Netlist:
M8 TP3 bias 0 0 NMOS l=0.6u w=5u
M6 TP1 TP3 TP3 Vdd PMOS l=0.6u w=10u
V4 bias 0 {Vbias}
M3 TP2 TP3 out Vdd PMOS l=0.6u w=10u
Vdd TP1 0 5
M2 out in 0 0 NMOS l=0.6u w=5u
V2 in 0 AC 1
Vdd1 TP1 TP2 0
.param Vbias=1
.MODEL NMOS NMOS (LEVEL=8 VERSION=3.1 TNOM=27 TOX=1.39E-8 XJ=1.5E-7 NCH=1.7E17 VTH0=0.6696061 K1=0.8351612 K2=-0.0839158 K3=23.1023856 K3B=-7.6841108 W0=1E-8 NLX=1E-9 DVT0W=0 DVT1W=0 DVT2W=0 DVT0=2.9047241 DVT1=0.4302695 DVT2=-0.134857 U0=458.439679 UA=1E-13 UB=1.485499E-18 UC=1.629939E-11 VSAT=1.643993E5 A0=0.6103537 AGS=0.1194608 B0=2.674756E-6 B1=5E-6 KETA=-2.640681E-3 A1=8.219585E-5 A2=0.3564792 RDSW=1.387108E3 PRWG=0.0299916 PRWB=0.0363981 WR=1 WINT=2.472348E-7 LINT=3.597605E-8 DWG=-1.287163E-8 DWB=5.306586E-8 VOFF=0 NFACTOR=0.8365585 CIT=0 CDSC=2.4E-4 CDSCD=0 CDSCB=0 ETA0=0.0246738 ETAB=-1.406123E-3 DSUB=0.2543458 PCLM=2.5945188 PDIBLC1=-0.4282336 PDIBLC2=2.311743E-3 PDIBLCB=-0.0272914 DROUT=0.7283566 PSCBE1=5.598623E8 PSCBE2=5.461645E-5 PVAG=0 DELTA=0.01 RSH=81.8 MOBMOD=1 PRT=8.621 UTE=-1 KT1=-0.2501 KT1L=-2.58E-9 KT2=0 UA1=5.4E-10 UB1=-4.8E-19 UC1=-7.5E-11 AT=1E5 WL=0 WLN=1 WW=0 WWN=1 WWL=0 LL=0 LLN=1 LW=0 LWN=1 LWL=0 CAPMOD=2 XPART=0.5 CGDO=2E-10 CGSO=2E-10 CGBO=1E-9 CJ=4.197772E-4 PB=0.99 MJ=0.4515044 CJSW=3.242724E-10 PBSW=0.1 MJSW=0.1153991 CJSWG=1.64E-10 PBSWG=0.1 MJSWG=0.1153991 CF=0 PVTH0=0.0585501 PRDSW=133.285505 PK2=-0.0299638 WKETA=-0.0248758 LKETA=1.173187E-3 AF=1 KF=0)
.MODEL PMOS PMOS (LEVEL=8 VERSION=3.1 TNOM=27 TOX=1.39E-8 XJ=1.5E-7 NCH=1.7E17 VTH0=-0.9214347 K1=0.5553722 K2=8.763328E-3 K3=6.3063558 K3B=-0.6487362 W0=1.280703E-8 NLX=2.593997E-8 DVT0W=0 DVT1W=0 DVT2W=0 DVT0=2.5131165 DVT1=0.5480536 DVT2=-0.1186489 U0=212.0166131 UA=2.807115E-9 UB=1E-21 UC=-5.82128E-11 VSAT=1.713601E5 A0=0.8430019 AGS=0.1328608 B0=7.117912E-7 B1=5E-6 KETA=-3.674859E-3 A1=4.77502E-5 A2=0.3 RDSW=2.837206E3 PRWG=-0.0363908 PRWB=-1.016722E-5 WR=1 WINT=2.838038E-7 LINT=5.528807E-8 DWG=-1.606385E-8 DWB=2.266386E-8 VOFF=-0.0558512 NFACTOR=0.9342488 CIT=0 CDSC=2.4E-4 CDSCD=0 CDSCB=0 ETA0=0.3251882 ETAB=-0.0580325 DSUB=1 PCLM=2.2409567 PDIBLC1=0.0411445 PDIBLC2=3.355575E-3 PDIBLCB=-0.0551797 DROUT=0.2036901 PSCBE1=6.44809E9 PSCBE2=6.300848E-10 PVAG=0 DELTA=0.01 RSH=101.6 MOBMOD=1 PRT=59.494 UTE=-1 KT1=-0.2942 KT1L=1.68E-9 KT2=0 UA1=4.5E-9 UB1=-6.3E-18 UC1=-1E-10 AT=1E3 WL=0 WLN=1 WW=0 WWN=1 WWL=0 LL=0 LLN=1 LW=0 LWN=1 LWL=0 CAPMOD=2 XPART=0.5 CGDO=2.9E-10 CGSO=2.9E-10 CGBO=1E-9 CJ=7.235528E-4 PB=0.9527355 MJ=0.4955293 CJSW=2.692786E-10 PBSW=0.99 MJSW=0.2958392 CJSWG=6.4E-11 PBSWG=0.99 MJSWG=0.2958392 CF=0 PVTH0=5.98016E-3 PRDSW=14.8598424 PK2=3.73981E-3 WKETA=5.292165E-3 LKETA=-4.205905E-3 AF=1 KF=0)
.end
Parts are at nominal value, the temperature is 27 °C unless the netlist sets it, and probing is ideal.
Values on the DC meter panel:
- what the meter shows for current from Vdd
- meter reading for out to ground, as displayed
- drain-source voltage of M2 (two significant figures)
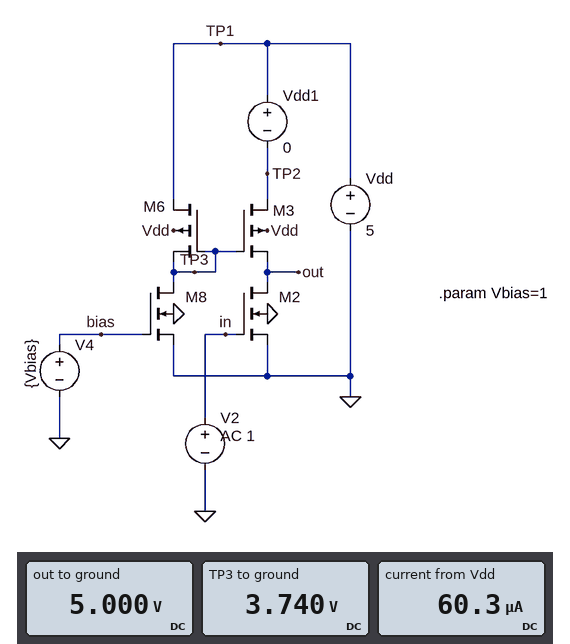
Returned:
60.3 µA
5.000 V
5.0 V
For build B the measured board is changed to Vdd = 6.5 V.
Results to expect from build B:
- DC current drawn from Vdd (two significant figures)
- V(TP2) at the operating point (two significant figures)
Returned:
71 µA
6.5 V
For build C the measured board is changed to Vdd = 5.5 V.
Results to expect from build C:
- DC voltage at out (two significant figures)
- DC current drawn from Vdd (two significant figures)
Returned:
5.5 V
63 µA
